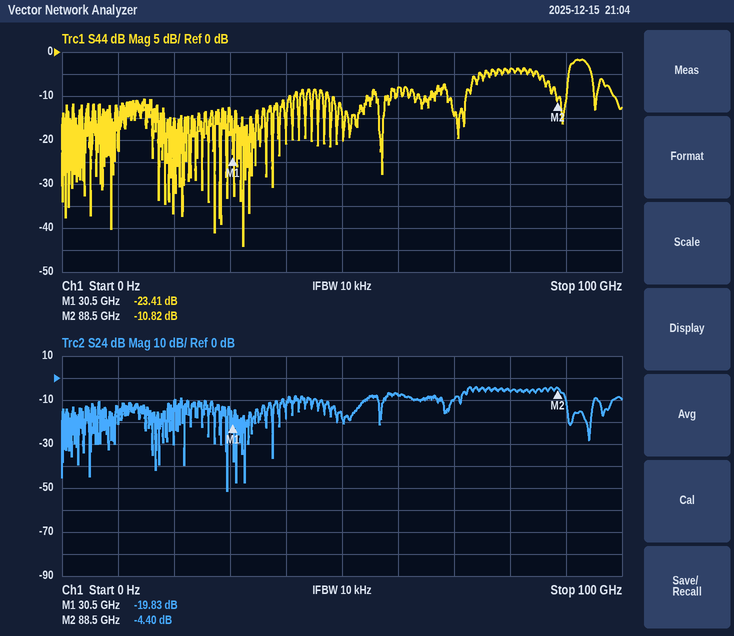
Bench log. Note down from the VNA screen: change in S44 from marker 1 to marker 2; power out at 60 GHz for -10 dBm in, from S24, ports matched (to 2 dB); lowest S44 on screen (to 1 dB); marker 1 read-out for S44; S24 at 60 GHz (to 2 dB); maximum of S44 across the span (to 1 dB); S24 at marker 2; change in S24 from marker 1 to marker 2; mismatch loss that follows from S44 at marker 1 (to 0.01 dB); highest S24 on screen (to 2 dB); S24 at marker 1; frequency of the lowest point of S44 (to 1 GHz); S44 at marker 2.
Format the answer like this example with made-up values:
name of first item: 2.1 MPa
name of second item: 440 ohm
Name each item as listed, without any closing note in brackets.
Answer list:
change in S44 from marker 1 to marker 2: 12.59 dB
power out at 60 GHz for -10 dBm in, from S24, ports matched: -18 dBm
lowest S44 on screen: -44 dB
marker 1 read-out for S44: -23.41 dB
S24 at 60 GHz: -8 dB
maximum of S44 across the span: -2 dB
S24 at marker 2: -4.40 dB
change in S24 from marker 1 to marker 2: 15.43 dB
mismatch loss that follows from S44 at marker 1: 0.02 dB
highest S24 on screen: -4 dB
S24 at marker 1: -19.83 dB
frequency of the lowest point of S44: 32 GHz
S44 at marker 2: -10.82 dB
